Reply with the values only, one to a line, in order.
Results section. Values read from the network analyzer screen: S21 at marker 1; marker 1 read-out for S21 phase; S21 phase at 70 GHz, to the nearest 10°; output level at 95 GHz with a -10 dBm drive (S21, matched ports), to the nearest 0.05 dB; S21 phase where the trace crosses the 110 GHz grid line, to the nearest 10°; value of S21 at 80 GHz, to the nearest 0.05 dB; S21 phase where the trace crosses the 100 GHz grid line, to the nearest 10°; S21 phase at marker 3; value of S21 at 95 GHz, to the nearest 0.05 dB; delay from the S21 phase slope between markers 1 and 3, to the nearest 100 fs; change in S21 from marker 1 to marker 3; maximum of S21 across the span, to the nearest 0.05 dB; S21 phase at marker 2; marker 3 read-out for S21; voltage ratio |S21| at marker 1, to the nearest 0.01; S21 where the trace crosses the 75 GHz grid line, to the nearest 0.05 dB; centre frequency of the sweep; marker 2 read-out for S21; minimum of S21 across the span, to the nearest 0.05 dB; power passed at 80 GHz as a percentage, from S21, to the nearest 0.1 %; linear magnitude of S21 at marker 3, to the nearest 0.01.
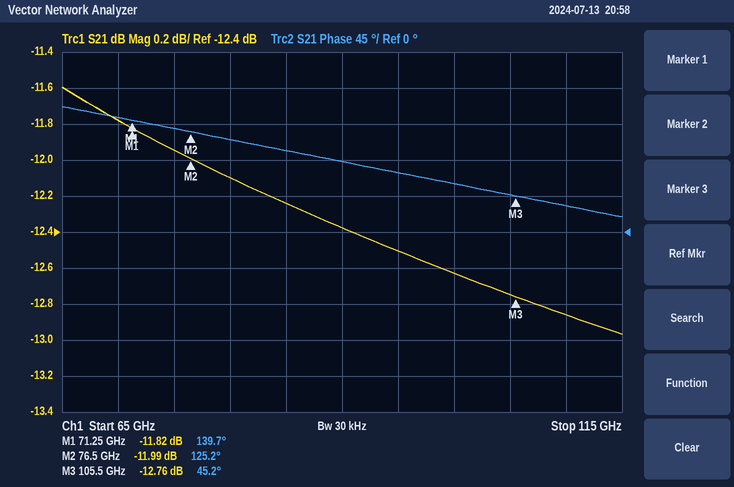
-11.82 dB
139.7°
140°
-22.50 dBm
30°
-12.10 dB
60°
45.2°
-12.50 dB
7.7 ps
-0.94 dB
-11.60 dB
125.2°
-12.76 dB
0.26
-11.95 dB
90 GHz
-11.99 dB
-12.95 dB
6.2 %
0.23
